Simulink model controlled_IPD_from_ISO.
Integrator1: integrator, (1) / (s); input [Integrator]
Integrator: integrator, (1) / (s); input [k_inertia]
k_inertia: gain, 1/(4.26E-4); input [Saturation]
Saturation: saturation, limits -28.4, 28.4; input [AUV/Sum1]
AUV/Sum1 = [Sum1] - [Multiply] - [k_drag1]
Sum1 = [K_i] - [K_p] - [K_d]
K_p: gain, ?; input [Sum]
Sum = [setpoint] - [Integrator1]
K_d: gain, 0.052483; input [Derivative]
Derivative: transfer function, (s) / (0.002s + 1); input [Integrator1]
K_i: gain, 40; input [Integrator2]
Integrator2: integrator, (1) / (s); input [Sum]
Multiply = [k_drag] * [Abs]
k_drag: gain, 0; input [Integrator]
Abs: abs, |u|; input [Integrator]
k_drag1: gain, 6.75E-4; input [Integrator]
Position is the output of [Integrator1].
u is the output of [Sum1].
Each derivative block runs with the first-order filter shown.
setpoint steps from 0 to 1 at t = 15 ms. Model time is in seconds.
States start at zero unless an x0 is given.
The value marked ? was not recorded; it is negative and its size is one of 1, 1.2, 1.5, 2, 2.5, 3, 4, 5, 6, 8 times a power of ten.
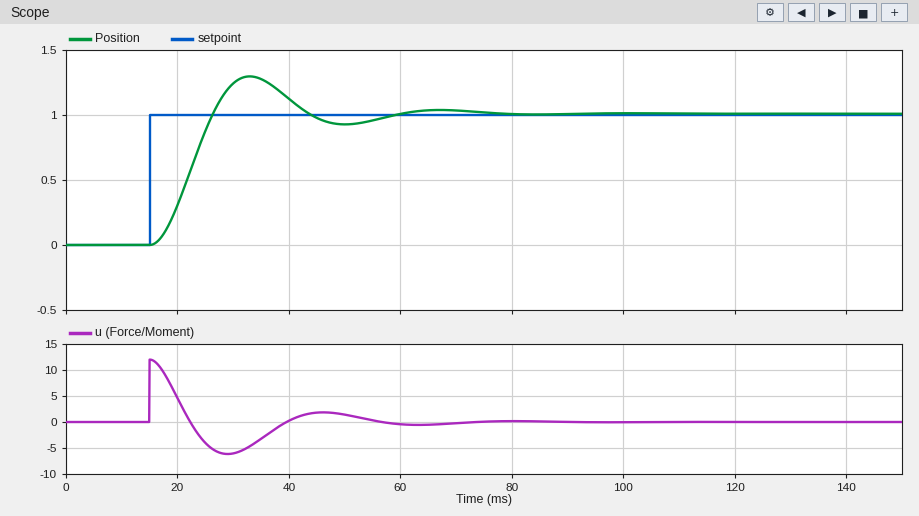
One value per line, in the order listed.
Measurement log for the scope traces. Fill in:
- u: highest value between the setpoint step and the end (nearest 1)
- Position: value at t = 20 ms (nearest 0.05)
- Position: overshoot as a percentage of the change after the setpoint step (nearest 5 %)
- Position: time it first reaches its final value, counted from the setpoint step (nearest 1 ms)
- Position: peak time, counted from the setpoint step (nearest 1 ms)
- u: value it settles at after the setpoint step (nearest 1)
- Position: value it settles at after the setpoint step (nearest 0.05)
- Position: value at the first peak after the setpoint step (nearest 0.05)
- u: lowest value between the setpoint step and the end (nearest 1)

12
0.30
30 %
11 ms
18 ms
0
1.00
1.30
-6
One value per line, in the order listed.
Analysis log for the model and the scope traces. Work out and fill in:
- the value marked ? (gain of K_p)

-12
